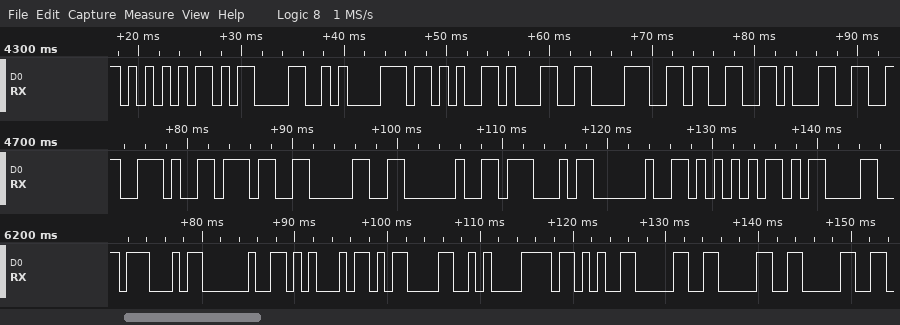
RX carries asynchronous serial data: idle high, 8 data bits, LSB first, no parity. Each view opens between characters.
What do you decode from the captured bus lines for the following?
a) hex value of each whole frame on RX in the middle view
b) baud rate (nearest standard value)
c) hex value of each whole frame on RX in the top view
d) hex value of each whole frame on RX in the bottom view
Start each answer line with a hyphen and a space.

- 2E, 37, 30, 20, 47, 20, 55, 0D
- 1200 baud
- 55, 0D, 0A, 2B, 31, 38, 33, 31
- 47, 20, 45, 0D, 0A, 2B, 30, 30, 30
